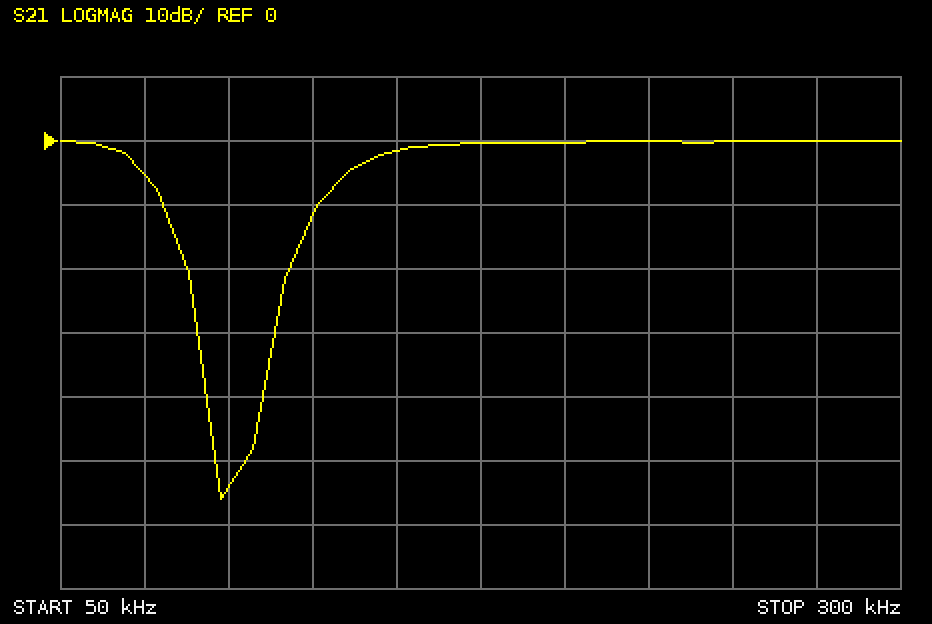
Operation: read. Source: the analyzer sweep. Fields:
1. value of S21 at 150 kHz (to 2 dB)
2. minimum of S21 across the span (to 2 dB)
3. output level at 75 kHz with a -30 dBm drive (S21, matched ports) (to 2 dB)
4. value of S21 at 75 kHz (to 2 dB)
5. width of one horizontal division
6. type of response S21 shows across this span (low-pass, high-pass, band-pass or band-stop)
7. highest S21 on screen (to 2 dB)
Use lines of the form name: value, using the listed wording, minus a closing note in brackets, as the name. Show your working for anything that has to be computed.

value of S21 at 150 kHz: -2 dB
minimum of S21 across the span: -56 dB
output level at 75 kHz with a -30 dBm drive (S21, matched ports): -30 dBm + (-6 dB) = -36 dBm
value of S21 at 75 kHz: -6 dB
width of one horizontal division: 25 kHz
type of response S21 shows across this span: band-stop
highest S21 on screen: 0 dB
